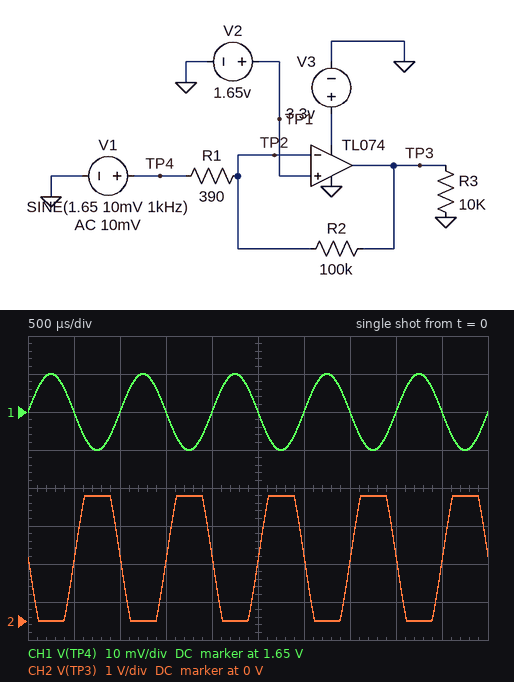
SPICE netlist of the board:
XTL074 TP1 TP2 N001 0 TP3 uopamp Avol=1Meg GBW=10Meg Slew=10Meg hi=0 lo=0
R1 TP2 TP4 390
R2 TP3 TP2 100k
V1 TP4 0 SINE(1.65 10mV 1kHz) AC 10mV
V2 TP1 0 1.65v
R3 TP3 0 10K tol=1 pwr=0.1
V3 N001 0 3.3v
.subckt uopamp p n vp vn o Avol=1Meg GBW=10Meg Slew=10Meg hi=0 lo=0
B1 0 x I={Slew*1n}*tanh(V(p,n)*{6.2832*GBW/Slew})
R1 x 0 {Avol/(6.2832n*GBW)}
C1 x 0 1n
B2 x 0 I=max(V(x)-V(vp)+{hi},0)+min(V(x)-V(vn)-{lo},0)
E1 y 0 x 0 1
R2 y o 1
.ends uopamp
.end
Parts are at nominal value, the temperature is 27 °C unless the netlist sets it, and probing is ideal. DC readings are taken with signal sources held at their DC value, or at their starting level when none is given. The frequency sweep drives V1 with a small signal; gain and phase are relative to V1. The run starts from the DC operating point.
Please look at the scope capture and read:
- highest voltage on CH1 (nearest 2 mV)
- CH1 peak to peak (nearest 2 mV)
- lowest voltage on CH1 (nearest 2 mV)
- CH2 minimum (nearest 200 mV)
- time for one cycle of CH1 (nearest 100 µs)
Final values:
1.660 V
20 mV
1.640 V
0 V
1.0 ms
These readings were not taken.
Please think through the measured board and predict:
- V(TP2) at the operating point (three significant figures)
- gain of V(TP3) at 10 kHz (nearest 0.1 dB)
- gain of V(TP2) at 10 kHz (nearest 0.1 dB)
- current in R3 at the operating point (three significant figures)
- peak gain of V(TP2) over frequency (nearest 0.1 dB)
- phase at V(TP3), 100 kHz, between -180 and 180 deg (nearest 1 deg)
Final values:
1.65 V
47.9 dB
-12.1 dB
165 µA
0 dB
111 deg
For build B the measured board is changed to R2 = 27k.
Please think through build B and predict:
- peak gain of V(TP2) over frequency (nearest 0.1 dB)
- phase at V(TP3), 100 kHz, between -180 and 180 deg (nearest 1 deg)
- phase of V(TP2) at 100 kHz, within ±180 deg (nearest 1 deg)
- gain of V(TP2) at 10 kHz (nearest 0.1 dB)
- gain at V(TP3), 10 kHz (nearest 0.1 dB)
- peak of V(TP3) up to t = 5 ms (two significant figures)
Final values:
-0.1 dB
145 deg
55 deg
-23.2 dB
36.8 dB
2.3 V
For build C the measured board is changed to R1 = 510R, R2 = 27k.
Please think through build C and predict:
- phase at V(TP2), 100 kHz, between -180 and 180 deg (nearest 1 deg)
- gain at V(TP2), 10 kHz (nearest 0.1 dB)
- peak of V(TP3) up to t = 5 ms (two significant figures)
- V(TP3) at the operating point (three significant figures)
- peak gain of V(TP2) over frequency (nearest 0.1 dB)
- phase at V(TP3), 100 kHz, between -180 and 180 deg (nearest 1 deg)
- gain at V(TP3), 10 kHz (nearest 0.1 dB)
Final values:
62 deg
-25.5 dB
2.2 V
1.65 V
-0.2 dB
152 deg
34.5 dB
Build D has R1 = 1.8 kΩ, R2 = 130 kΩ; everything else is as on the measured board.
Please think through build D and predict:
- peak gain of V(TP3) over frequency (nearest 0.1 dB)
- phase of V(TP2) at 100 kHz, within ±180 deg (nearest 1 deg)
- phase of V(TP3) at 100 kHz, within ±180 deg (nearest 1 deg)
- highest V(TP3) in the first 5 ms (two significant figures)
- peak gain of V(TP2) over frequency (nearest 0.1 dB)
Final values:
37.2 dB
54 deg
144 deg
2.4 V
-0.1 dB
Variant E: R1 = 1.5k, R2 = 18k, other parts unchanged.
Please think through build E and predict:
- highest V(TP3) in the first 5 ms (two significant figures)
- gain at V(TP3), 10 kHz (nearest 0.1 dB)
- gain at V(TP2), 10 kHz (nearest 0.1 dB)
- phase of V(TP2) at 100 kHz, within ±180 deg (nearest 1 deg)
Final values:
1.8 V
21.6 dB
-38.4 dB
83 deg
